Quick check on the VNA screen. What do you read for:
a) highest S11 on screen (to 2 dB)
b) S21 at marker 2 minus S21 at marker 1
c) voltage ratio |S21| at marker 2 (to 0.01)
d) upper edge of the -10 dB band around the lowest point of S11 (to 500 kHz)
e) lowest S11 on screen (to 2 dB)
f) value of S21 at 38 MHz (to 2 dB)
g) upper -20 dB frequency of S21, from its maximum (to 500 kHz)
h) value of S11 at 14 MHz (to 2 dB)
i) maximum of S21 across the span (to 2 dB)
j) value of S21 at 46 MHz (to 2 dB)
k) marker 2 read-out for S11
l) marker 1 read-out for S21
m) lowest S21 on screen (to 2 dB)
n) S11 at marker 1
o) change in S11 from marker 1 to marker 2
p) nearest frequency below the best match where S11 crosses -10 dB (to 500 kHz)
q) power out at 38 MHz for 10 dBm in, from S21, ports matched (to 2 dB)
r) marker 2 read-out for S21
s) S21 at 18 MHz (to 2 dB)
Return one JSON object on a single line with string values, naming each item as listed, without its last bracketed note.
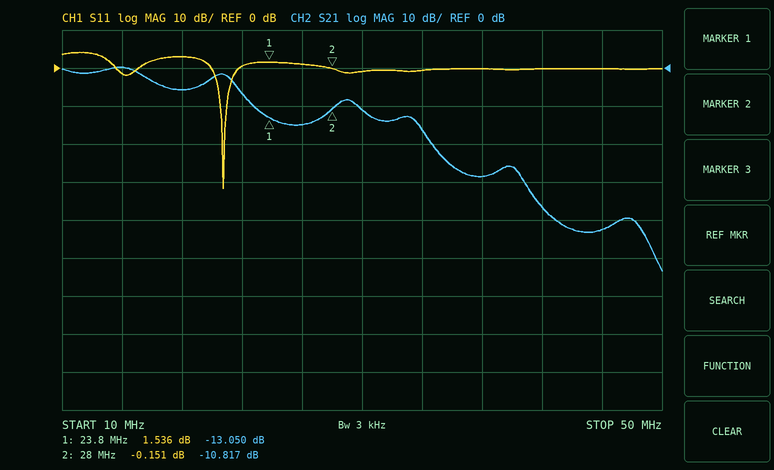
{"highest S11 on screen": "4 dB", "S21 at marker 2 minus S21 at marker 1": "2.233 dB", "voltage ratio |S21| at marker 2": "0.29", "upper edge of the -10 dB band around the lowest point of S11": "21.0 MHz", "lowest S11 on screen": "-32 dB", "value of S21 at 38 MHz": "-28 dB", "upper -20 dB frequency of S21, from its maximum": "34.5 MHz", "value of S11 at 14 MHz": "-2 dB", "maximum of S21 across the span": "0 dB", "value of S21 at 46 MHz": "-42 dB", "marker 2 read-out for S11": "-0.151 dB", "marker 1 read-out for S21": "-13.050 dB", "lowest S21 on screen": "-54 dB", "S11 at marker 1": "1.536 dB", "change in S11 from marker 1 to marker 2": "-1.687 dB", "nearest frequency below the best match where S11 crosses -10 dB": "20.5 MHz", "power out at 38 MHz for 10 dBm in, from S21, ports matched": "-18 dBm", "marker 2 read-out for S21": "-10.817 dB", "S21 at 18 MHz": "-6 dB"}
